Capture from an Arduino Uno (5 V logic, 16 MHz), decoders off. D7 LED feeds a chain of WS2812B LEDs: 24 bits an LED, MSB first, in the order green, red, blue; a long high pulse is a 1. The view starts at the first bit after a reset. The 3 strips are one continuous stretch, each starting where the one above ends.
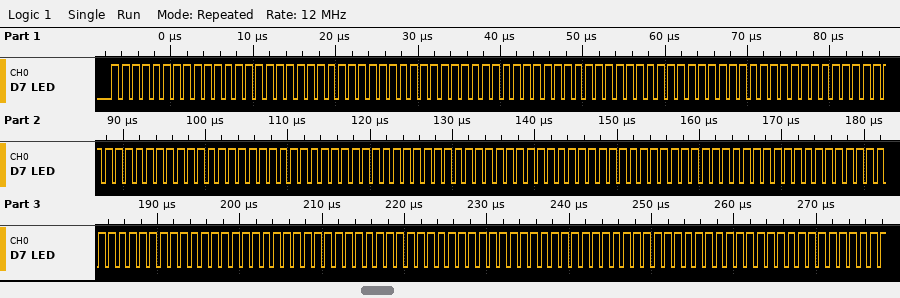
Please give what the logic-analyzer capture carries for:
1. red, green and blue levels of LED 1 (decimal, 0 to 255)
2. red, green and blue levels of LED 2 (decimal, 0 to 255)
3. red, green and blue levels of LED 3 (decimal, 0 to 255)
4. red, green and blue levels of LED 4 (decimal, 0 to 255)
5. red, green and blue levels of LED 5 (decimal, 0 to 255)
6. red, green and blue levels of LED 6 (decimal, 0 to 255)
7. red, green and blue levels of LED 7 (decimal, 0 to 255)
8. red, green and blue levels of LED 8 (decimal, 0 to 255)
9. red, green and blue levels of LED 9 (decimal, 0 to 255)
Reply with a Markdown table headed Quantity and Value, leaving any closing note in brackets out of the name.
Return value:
| Quantity | Value |
|---|---|
| red, green and blue levels of LED 1 | 255, 255, 255 |
| red, green and blue levels of LED 2 | 255, 255, 255 |
| red, green and blue levels of LED 3 | 255, 255, 255 |
| red, green and blue levels of LED 4 | 255, 255, 255 |
| red, green and blue levels of LED 5 | 255, 255, 255 |
| red, green and blue levels of LED 6 | 255, 255, 255 |
| red, green and blue levels of LED 7 | 255, 255, 255 |
| red, green and blue levels of LED 8 | 255, 255, 255 |
| red, green and blue levels of LED 9 | 255, 255, 255 |
